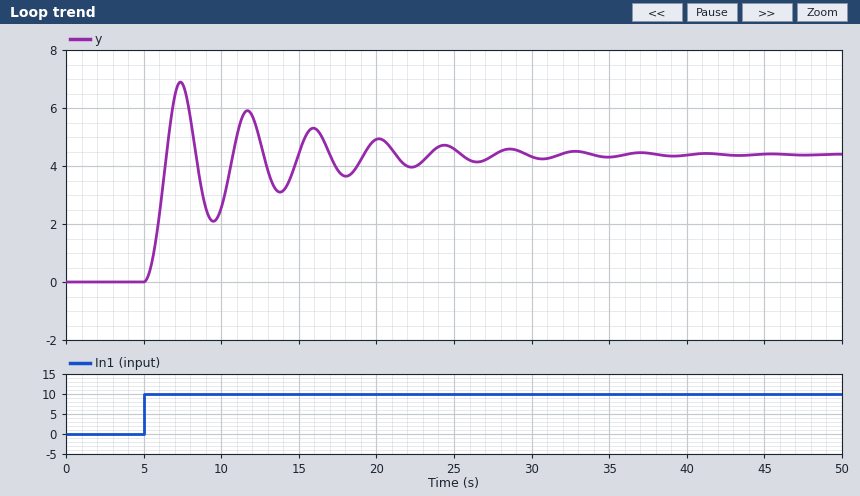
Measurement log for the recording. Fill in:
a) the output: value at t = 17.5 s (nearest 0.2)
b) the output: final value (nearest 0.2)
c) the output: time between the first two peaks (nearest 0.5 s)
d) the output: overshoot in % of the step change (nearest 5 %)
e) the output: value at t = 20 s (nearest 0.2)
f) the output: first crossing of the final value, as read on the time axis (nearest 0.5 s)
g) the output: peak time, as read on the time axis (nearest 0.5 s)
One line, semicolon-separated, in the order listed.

3.8; 4.4; 4.5 s; 55 %; 5.0; 6.5 s; 7.5 s
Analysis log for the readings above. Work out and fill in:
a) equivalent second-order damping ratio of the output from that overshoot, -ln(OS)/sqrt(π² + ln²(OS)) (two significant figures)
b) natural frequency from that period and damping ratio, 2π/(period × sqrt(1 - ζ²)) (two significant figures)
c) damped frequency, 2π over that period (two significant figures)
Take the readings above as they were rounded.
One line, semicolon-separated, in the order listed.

0.19; 1.4 rad/s; 1.4 rad/s
